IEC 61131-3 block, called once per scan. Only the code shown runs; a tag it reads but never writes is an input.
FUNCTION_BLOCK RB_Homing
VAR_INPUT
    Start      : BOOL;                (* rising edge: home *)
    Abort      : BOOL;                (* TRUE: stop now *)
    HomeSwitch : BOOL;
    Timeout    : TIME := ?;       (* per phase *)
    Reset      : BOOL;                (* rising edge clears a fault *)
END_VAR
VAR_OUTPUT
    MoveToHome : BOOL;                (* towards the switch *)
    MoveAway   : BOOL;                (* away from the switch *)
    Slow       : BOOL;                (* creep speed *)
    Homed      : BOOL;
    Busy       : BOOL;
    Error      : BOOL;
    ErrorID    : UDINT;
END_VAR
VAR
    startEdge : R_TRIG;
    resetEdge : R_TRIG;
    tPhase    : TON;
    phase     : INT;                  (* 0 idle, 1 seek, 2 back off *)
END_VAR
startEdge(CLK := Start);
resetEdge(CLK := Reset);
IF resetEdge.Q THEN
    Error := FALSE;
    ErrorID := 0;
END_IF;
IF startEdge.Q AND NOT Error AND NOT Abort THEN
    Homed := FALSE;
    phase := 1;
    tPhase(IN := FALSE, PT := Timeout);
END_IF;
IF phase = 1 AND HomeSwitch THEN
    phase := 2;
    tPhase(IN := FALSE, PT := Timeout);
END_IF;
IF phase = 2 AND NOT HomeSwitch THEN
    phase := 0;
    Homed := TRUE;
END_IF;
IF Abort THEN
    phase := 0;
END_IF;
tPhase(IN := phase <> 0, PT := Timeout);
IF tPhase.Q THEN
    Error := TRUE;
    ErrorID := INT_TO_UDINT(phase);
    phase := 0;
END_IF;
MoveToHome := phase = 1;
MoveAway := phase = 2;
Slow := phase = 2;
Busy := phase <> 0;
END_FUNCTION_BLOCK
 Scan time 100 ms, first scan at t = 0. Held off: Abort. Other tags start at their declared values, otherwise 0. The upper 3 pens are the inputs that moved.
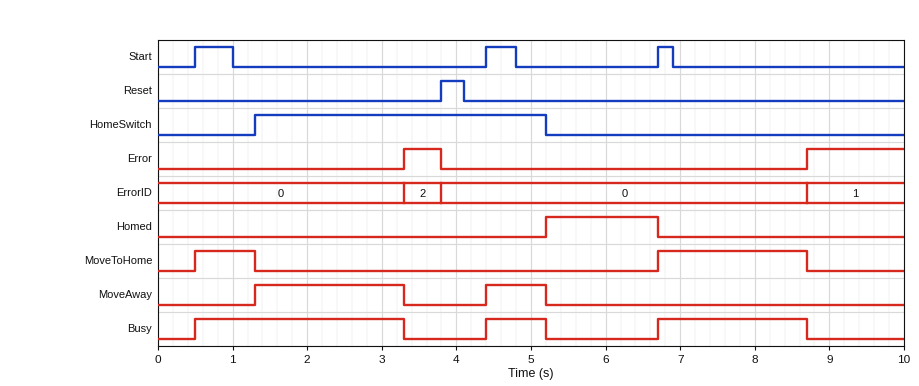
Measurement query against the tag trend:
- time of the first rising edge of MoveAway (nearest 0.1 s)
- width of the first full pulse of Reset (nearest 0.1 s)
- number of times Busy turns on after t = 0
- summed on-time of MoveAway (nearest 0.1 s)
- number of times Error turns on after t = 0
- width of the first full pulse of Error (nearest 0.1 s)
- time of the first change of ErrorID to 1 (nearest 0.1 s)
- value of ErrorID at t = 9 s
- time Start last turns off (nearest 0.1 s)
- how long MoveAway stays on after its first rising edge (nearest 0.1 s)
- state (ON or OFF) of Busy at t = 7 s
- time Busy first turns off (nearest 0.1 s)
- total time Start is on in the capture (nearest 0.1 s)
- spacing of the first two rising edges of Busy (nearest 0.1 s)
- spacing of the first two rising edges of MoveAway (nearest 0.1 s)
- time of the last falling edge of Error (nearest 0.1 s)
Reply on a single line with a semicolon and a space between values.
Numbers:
1.3 s; 0.3 s; 3; 2.8 s; 2; 0.5 s; 8.7 s; 1; 6.9 s; 2.0 s; ON; 3.3 s; 1.1 s; 3.9 s; 3.1 s; 3.8 s
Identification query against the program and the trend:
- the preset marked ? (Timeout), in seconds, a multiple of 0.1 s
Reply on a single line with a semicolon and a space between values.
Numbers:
2.0 s
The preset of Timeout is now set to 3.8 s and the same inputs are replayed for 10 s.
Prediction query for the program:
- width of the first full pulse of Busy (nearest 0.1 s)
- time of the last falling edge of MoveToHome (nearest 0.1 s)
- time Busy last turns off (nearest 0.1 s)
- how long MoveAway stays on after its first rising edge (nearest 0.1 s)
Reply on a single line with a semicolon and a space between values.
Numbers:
4.7 s; 1.3 s; 5.2 s; 3.9 s
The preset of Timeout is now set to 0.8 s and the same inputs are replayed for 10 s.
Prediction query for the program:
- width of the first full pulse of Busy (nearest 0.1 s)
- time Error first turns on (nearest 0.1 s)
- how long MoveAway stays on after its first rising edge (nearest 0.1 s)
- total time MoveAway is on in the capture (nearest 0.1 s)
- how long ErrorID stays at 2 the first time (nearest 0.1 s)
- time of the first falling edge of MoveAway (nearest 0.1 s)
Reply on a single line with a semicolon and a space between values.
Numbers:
1.6 s; 2.1 s; 0.8 s; 1.6 s; 1.7 s; 2.1 s
